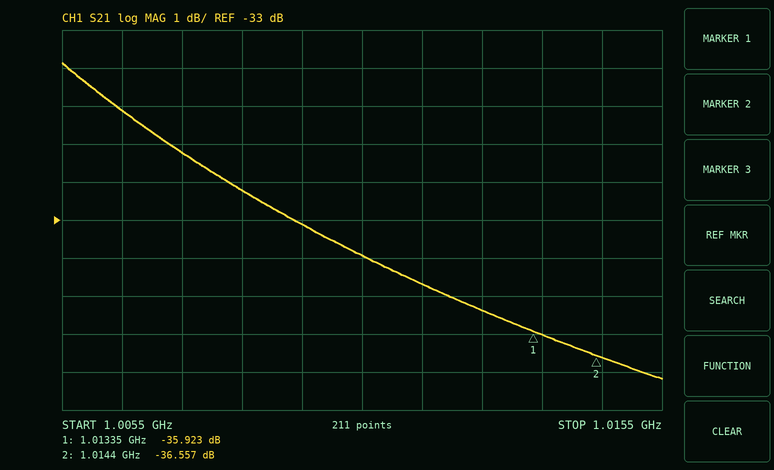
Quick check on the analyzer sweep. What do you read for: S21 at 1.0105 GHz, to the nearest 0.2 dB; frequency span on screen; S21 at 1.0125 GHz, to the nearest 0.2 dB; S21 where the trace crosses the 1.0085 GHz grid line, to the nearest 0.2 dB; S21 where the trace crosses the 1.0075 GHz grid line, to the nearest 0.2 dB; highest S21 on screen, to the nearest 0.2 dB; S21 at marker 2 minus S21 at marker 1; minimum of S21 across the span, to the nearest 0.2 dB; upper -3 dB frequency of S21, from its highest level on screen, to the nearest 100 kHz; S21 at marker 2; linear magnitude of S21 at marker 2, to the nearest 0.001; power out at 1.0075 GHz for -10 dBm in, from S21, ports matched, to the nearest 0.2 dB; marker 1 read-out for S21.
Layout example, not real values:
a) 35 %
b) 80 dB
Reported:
a) -34.0 dB
b) 10 MHz
c) -35.4 dB
d) -32.2 dB
e) -31.2 dB
f) -28.8 dB
g) -0.634 dB
h) -37.2 dB
i) 1.0081 GHz
j) -36.557 dB
k) 0.015
l) -41.2 dBm
m) -35.923 dB
